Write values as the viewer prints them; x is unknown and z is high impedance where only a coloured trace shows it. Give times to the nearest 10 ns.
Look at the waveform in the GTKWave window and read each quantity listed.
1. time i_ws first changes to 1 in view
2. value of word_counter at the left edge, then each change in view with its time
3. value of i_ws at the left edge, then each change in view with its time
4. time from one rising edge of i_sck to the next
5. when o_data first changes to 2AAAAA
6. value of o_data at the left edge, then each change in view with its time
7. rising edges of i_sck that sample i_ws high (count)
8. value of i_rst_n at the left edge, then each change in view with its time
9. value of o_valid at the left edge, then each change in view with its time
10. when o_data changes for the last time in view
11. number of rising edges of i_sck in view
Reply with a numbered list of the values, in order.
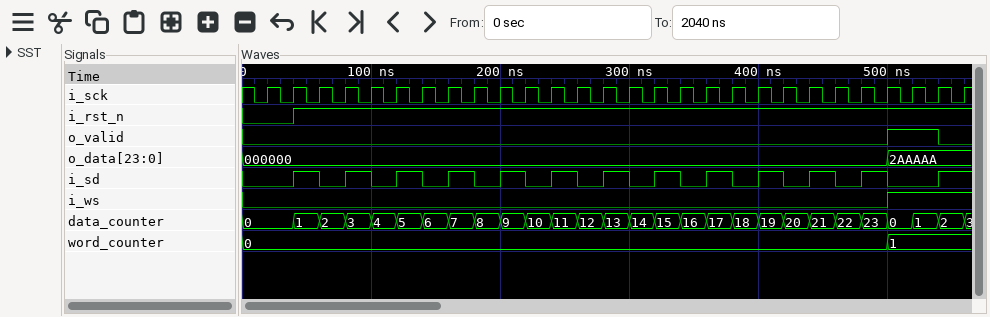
1. 500 ns
2. 0, 1 at 500 ns
3. 0, 1 at 500 ns
4. 20 ns
5. 500 ns
6. 000000, 2AAAAA at 500 ns
7. 3
8. 0, 1 at 40 ns
9. 0, 1 at 500 ns, 0 at 540 ns
10. 500 ns
11. 28
